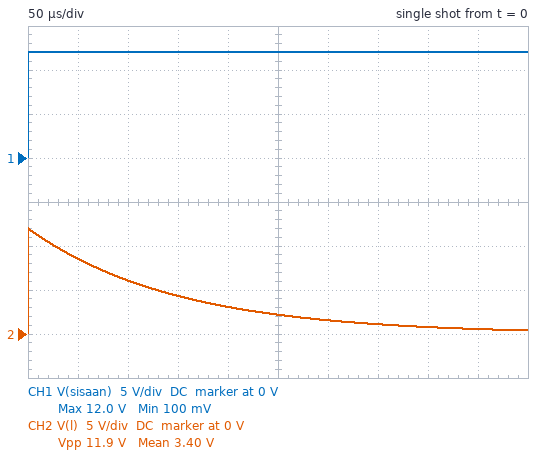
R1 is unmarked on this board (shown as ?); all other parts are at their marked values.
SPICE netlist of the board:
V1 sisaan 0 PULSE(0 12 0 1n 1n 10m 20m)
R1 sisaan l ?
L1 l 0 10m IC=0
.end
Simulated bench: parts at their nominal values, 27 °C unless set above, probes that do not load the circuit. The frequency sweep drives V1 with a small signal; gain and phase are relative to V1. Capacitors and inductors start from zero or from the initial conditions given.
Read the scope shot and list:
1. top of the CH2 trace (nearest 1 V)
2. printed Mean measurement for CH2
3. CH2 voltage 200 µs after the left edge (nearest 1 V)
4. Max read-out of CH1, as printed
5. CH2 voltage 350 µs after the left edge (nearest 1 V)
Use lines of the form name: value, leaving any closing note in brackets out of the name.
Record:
top of the CH2 trace: 12 V
printed Mean measurement for CH2: 3.40 V
CH2 voltage 200 µs after the left edge: 3 V
Max read-out of CH1, as printed: 12.0 V
CH2 voltage 350 µs after the left edge: 1 V
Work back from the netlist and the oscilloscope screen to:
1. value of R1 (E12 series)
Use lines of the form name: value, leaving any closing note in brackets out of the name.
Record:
value of R1: 68 Ω
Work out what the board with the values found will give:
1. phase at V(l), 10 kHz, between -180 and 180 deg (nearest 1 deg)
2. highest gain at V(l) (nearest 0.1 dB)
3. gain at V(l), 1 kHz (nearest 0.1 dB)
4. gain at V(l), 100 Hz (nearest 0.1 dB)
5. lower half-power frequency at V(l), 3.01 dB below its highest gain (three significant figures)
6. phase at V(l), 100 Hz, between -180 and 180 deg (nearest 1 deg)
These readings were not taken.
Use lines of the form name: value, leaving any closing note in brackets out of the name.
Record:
phase at V(l), 10 kHz, between -180 and 180 deg: 6 deg
highest gain at V(l): 0 dB
gain at V(l), 1 kHz: -3.4 dB
gain at V(l), 100 Hz: -20.7 dB
lower half-power frequency at V(l), 3.01 dB below its highest gain: 1.08 kHz
phase at V(l), 100 Hz, between -180 and 180 deg: 85 deg
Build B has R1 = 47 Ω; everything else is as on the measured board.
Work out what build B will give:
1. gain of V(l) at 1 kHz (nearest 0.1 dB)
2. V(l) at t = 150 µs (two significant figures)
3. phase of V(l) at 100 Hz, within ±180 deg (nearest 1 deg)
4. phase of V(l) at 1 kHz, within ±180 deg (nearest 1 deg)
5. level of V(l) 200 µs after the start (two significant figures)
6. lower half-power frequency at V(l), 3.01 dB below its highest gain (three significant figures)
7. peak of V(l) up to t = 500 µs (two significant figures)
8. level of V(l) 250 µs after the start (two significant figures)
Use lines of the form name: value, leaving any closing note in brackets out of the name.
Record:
gain of V(l) at 1 kHz: -1.9 dB
V(l) at t = 150 µs: 5.9 V
phase of V(l) at 100 Hz, within ±180 deg: 82 deg
phase of V(l) at 1 kHz, within ±180 deg: 37 deg
level of V(l) 200 µs after the start: 4.7 V
lower half-power frequency at V(l), 3.01 dB below its highest gain: 748 Hz
peak of V(l) up to t = 500 µs: 12 V
level of V(l) 250 µs after the start: 3.7 V
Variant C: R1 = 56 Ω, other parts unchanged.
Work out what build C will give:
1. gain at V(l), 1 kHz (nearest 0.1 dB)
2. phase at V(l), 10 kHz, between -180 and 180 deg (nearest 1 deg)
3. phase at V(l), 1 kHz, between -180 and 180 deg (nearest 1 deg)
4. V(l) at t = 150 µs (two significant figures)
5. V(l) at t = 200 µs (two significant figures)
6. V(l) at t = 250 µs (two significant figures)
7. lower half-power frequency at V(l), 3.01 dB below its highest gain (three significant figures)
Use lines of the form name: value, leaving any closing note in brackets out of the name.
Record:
gain at V(l), 1 kHz: -2.5 dB
phase at V(l), 10 kHz, between -180 and 180 deg: 5 deg
phase at V(l), 1 kHz, between -180 and 180 deg: 42 deg
V(l) at t = 150 µs: 5.2 V
V(l) at t = 200 µs: 3.9 V
V(l) at t = 250 µs: 3.0 V
lower half-power frequency at V(l), 3.01 dB below its highest gain: 891 Hz
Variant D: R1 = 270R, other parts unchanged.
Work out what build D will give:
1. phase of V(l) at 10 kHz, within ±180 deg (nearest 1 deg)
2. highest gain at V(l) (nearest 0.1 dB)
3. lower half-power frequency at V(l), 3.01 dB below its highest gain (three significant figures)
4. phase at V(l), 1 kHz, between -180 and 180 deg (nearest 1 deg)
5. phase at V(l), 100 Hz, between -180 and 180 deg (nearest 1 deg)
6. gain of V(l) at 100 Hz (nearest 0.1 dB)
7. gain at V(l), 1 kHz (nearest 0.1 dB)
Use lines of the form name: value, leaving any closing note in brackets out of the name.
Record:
phase of V(l) at 10 kHz, within ±180 deg: 23 deg
highest gain at V(l): 0 dB
lower half-power frequency at V(l), 3.01 dB below its highest gain: 4.30 kHz
phase at V(l), 1 kHz, between -180 and 180 deg: 77 deg
phase at V(l), 100 Hz, between -180 and 180 deg: 89 deg
gain of V(l) at 100 Hz: -32.7 dB
gain at V(l), 1 kHz: -12.9 dB
